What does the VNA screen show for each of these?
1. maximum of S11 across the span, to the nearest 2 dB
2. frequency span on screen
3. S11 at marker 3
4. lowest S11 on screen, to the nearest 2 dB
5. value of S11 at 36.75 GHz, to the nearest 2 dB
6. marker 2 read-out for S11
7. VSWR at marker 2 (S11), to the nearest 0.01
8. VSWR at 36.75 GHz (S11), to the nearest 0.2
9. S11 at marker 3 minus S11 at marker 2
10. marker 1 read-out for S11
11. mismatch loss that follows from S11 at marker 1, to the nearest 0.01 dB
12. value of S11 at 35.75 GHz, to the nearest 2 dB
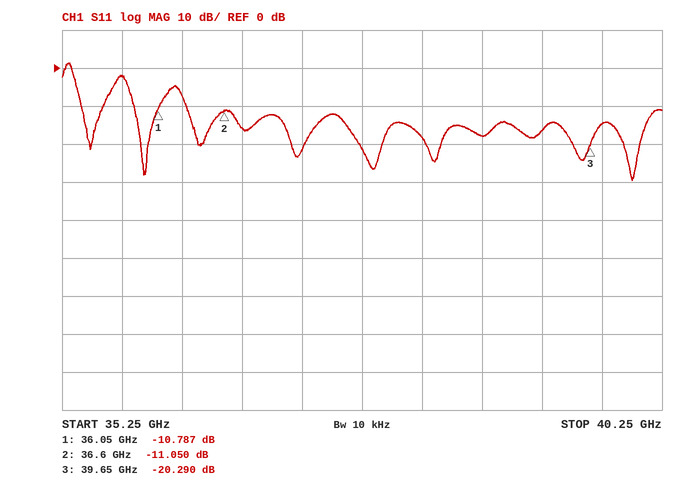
2 dB
5 GHz
-20.290 dB
-30 dB
-16 dB
-11.050 dB
1.78
1.4
-9.240 dB
-10.787 dB
0.38 dB
-2 dB
